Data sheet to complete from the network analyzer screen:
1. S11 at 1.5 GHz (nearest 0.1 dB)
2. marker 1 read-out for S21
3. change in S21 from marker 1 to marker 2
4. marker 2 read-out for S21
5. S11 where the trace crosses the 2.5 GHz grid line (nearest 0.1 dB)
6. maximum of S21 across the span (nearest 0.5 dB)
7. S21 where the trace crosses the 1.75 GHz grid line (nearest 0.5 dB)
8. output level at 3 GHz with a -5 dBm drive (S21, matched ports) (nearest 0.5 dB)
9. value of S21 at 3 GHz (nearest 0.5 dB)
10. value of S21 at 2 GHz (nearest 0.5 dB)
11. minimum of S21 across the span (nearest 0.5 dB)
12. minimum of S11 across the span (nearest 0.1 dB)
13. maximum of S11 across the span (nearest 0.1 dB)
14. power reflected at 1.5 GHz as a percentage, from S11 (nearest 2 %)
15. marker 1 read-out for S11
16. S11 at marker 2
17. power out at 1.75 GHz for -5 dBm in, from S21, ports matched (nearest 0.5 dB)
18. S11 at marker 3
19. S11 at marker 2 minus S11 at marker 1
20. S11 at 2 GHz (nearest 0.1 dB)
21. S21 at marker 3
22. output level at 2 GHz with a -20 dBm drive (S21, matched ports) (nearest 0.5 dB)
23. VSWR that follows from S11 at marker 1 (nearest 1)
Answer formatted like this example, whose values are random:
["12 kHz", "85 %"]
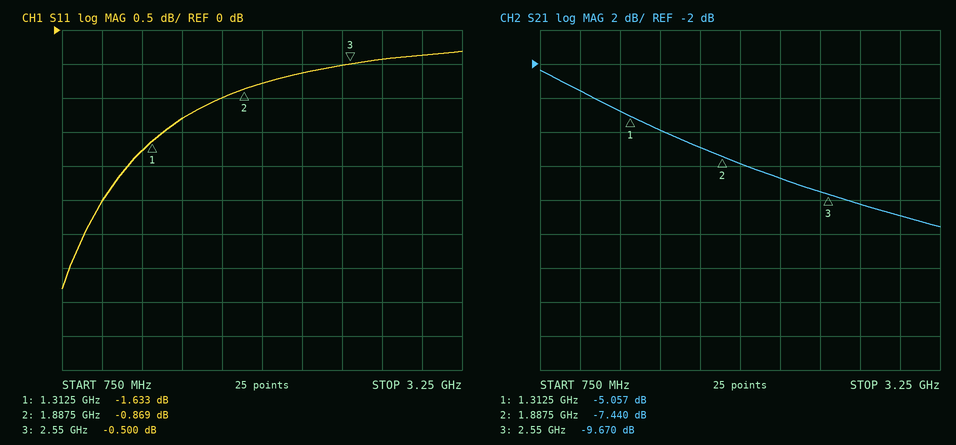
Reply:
["-1.3 dB", "-5.057 dB", "-2.383 dB", "-7.440 dB", "-0.5 dB", "-2.5 dB", "-7.0 dB", "-16.0 dBm", "-11.0 dB", "-8.0 dB", "-11.5 dB", "-3.8 dB", "-0.3 dB", "74 %", "-1.633 dB", "-0.869 dB", "-12.0 dBm", "-0.500 dB", "0.764 dB", "-0.8 dB", "-9.670 dB", "-28.0 dBm", "11"]
